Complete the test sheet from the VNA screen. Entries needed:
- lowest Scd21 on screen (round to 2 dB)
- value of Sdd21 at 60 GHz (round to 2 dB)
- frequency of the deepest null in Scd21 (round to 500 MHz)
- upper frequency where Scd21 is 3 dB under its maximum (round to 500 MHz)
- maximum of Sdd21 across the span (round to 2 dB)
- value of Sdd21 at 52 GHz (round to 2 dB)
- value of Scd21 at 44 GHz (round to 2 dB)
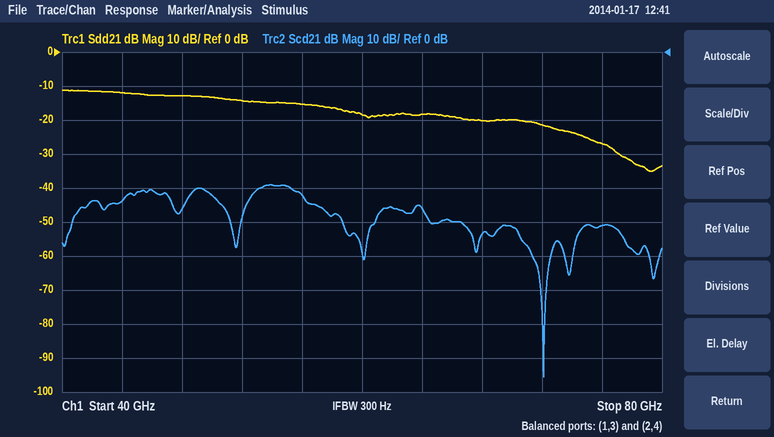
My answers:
-96 dB
-18 dB
72.0 GHz
56.0 GHz
-12 dB
-14 dB
-44 dB
